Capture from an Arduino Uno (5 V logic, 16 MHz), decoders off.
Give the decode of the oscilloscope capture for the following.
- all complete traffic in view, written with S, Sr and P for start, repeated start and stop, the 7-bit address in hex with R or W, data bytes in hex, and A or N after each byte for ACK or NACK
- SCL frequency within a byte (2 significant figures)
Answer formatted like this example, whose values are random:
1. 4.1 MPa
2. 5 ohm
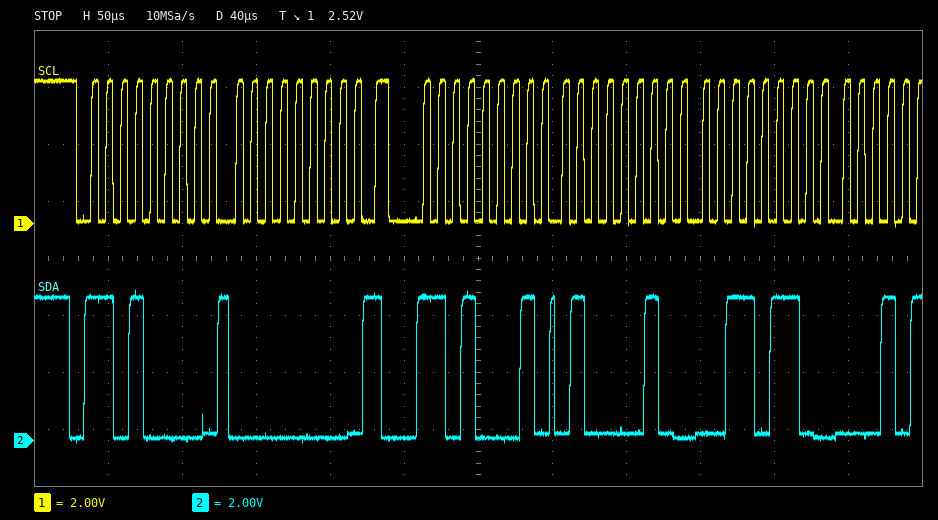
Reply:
1. S 68W A 00 A Sr 68R A 42 A 36 A
2. 100 kHz
